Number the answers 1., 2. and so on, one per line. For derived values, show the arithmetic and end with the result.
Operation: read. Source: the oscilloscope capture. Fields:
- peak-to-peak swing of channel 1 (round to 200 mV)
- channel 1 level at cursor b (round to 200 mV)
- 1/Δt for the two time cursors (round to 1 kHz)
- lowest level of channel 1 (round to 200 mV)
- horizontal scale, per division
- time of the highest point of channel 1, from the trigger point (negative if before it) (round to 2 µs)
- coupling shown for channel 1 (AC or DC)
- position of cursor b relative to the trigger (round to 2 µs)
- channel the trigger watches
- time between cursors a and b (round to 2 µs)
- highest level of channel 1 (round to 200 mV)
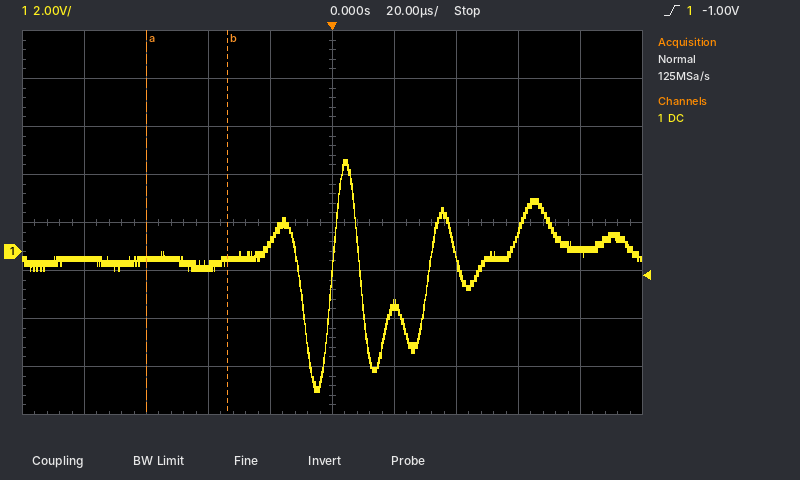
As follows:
1. 3.8 V − (-5.8 V) = 9.6 V
2. -400 mV
3. 1 / 26 µs ≈ 38 kHz
4. -5.8 V
5. 20 µs
6. +4 µs
7. DC
8. -34 µs
9. channel 1
10. 26 µs
11. 3.8 V
